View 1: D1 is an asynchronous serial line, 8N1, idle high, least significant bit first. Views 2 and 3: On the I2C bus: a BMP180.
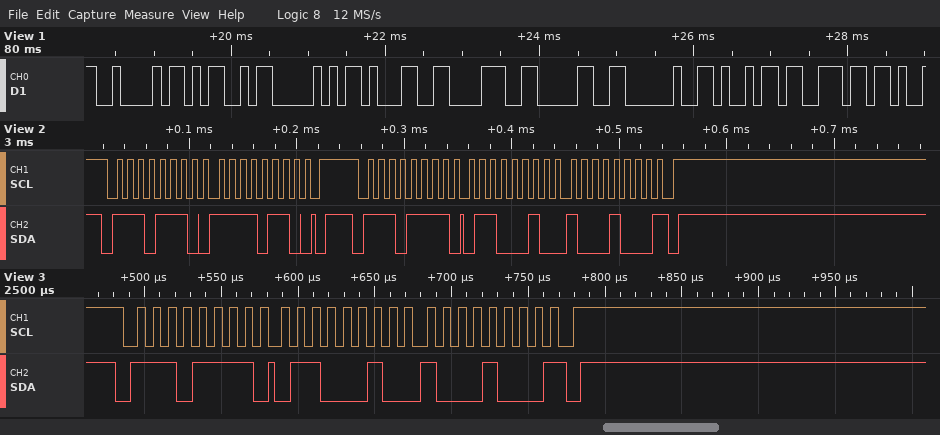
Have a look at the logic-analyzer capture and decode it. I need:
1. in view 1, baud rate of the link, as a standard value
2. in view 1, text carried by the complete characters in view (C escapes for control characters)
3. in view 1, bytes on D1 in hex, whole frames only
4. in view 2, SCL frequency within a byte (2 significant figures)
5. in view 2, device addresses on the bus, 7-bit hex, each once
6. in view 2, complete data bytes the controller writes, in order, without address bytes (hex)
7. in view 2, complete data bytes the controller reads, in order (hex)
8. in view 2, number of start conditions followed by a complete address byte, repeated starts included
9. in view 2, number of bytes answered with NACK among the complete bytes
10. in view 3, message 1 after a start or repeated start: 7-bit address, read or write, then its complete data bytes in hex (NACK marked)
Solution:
9600 baud
"BMP180 in"
42 4D 50 31 38 30 20 69 6E
100 kHz
0x77
F6
62 88
2
1
0x77 read: 62 88 NACK
